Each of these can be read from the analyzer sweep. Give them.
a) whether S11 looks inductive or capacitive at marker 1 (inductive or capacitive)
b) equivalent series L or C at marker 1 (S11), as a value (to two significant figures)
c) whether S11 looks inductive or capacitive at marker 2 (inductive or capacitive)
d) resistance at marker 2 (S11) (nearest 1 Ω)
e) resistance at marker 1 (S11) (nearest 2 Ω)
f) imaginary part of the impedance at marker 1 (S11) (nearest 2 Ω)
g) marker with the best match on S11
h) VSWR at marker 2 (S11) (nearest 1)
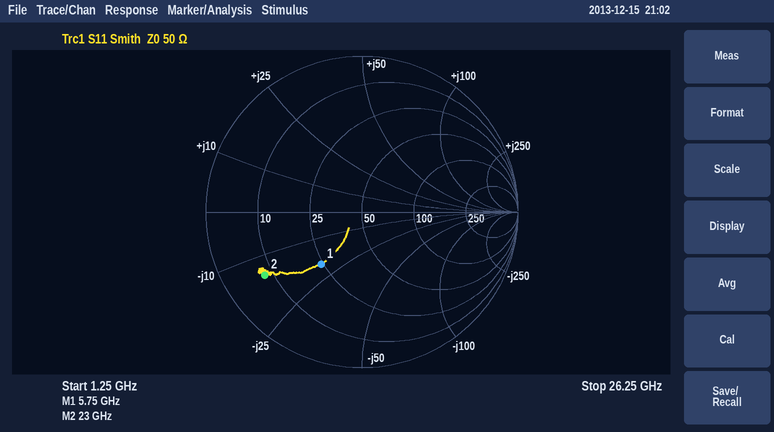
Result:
capacitive
1.4 pF
capacitive
8 Ω
24 Ω
-20 Ω
marker 1
7
